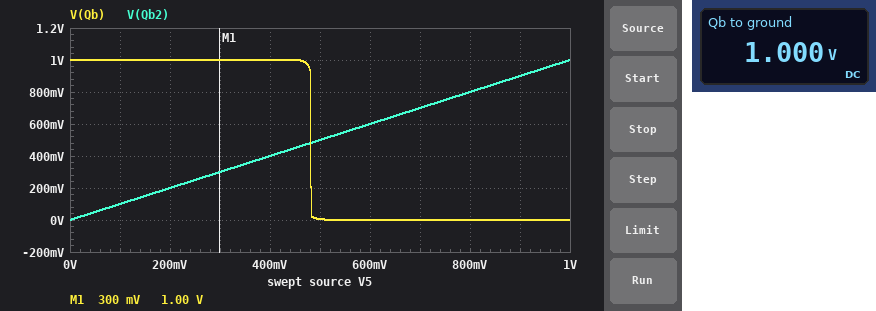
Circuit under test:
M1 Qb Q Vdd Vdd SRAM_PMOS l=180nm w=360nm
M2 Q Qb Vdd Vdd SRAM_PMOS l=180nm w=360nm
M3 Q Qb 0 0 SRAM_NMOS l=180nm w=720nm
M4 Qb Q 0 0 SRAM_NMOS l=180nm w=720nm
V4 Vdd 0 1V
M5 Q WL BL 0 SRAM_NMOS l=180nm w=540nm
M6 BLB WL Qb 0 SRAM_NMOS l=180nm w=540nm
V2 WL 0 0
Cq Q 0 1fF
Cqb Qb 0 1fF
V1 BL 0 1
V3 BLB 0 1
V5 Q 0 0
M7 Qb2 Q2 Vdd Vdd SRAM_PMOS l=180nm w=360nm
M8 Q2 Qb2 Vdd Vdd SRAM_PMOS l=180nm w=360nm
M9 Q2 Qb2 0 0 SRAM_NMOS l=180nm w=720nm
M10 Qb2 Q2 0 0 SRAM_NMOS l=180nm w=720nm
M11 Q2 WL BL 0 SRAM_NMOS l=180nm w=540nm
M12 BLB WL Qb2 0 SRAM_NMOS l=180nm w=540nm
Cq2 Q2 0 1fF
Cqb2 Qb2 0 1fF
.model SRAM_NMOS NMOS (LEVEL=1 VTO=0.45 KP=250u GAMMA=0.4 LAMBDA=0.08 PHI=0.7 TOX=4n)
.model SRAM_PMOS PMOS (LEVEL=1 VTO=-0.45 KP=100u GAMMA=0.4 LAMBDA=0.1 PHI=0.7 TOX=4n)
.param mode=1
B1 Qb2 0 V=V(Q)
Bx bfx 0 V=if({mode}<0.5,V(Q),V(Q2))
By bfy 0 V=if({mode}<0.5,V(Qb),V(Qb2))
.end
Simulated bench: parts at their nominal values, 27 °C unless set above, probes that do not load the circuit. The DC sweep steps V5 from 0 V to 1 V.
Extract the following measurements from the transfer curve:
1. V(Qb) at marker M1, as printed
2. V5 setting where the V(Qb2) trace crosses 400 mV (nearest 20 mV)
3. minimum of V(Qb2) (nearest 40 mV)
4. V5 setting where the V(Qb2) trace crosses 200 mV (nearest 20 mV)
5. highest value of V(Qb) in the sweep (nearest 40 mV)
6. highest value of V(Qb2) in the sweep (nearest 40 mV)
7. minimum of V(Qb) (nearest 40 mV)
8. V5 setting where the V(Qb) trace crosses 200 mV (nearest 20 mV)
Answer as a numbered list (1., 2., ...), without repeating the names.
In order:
1. 1.00 V
2. 400 mV
3. 0 V
4. 200 mV
5. 1.00 V
6. 1.00 V
7. 0 V
8. 480 mV
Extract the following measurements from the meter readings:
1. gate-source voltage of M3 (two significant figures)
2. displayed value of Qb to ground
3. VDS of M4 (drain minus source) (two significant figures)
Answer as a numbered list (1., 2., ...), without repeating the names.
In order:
1. 1.0 V
2. 1.000 V
3. 1.0 V
